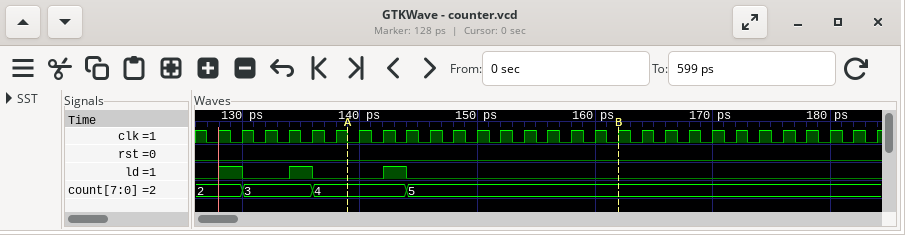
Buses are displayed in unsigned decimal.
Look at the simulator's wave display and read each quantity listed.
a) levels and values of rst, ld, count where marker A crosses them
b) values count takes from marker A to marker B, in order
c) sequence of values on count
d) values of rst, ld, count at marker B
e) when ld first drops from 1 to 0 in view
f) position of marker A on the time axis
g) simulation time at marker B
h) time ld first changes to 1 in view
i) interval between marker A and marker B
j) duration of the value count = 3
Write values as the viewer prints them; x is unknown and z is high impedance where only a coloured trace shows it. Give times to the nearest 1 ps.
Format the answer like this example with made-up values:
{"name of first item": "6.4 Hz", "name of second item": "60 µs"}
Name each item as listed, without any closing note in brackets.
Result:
{"levels and values of rst, ld, count where marker A crosses them": "rst=0, ld=0, count=4", "values count takes from marker A to marker B, in order": "4, 5", "sequence of values on count": "2, 3, 4, 5", "values of rst, ld, count at marker B": "rst=0, ld=0, count=5", "when ld first drops from 1 to 0 in view": "130 ps", "position of marker A on the time axis": "139 ps", "simulation time at marker B": "162 ps", "time ld first changes to 1 in view": "128 ps", "interval between marker A and marker B": "23 ps", "duration of the value count = 3": "6 ps"}
